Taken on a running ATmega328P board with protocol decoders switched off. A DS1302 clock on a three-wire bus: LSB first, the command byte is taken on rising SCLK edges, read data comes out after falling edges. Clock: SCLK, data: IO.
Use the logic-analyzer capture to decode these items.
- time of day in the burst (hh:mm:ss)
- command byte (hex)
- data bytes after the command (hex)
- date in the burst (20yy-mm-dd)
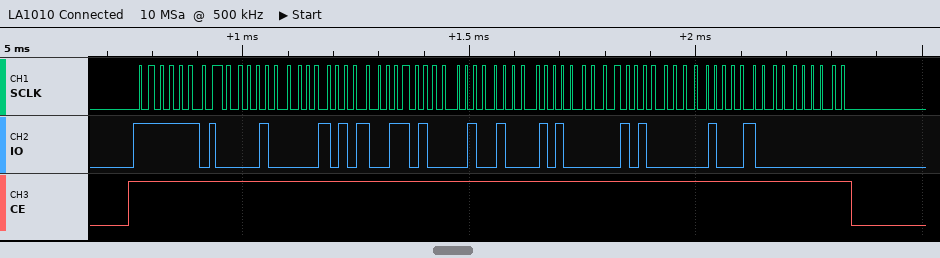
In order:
16:54:10
0xBF
10 54 16 12 05 05 22 00
2022-05-12
